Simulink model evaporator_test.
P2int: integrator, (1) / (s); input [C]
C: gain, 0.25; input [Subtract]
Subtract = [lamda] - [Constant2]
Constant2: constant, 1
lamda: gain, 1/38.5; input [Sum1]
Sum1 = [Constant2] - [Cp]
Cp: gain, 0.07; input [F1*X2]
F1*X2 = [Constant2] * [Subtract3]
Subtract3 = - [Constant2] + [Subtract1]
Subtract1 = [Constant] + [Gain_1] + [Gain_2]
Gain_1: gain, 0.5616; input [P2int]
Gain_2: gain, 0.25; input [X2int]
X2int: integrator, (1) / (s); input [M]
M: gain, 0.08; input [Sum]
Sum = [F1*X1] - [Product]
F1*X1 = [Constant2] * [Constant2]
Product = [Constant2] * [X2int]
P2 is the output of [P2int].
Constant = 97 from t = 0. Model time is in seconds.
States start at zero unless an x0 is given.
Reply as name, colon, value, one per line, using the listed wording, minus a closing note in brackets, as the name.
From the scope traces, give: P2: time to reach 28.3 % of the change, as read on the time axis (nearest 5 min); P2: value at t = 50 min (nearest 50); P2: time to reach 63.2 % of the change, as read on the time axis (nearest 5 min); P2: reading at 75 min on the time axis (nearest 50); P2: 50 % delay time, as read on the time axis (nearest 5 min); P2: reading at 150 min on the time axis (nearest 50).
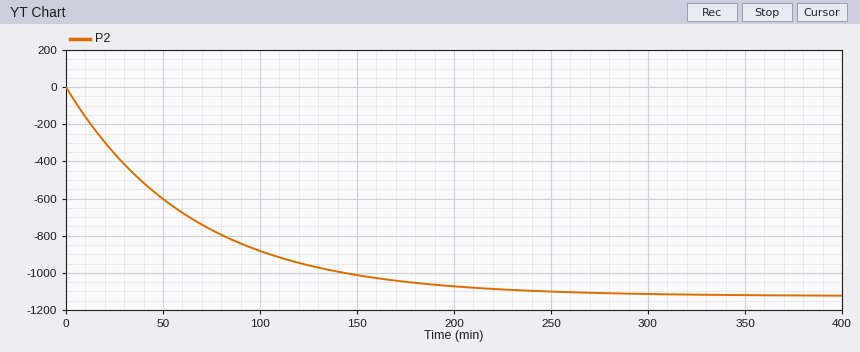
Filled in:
P2: time to reach 28.3 % of the change, as read on the time axis: 20 min
P2: value at t = 50 min: -600
P2: time to reach 63.2 % of the change, as read on the time axis: 65 min
P2: reading at 75 min on the time axis: -750
P2: 50 % delay time, as read on the time axis: 45 min
P2: reading at 150 min on the time axis: -1000
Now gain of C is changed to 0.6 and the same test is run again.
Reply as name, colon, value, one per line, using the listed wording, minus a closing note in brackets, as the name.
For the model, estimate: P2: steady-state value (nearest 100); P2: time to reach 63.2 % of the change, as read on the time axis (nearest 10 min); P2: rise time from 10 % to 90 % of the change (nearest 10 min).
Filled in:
P2: steady-state value: -1100
P2: time to reach 63.2 % of the change, as read on the time axis: 30 min
P2: rise time from 10 % to 90 % of the change: 60 min
